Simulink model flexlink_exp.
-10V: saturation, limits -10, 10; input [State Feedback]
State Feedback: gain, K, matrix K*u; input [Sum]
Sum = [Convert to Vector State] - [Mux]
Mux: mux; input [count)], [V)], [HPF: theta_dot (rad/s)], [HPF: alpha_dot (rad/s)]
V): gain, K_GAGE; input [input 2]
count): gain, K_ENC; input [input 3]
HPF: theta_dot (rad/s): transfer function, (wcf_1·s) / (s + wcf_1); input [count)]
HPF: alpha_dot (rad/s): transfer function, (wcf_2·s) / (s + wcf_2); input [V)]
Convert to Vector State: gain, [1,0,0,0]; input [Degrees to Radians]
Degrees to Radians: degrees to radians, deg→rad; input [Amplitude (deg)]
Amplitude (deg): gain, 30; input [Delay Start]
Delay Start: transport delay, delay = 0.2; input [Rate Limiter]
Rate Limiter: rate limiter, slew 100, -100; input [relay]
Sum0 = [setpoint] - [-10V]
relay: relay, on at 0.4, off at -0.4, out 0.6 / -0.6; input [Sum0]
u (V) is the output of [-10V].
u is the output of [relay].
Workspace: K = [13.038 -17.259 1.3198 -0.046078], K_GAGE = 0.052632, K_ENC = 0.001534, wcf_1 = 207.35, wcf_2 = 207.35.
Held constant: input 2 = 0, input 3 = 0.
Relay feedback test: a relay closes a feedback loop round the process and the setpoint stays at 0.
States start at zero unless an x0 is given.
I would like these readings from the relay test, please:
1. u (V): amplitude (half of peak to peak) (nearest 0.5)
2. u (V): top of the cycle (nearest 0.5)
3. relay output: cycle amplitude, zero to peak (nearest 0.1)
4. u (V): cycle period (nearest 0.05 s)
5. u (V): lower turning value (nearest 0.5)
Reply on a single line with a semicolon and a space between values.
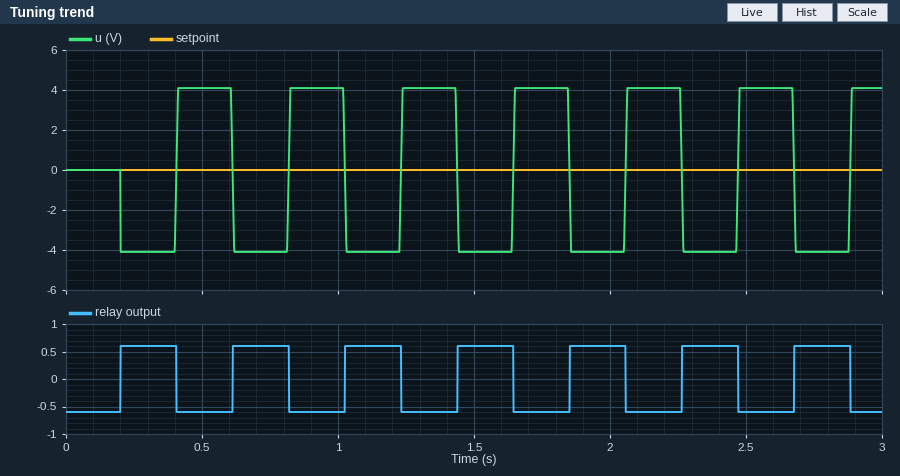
4.0; 4.0; 0.6; 0.40 s; -4.0
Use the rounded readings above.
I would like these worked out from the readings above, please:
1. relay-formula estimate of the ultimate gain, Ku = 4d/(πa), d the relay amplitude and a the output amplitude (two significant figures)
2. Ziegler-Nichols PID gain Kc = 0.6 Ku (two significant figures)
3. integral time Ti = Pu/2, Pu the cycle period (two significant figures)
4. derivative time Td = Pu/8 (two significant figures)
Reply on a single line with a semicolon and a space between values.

0.19; 0.11; 0.20 s; 0.050 s
